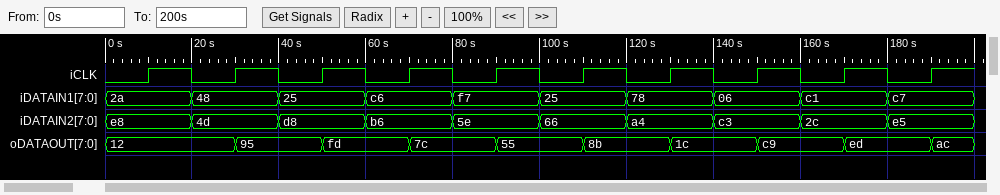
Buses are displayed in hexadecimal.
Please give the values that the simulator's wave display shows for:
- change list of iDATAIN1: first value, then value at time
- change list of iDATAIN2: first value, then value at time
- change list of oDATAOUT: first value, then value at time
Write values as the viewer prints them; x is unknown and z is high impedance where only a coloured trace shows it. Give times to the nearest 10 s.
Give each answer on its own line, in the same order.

2a, 48 at 20 s, 25 at 40 s, c6 at 60 s, f7 at 80 s, 25 at 100 s, 78 at 120 s, 06 at 140 s, c1 at 160 s, c7 at 180 s
e8, 4d at 20 s, d8 at 40 s, b6 at 60 s, 5e at 80 s, 66 at 100 s, a4 at 120 s, c3 at 140 s, 2c at 160 s, e5 at 180 s
12, 95 at 30 s, fd at 50 s, 7c at 70 s, 55 at 90 s, 8b at 110 s, 1c at 130 s, c9 at 150 s, ed at 170 s, ac at 190 s
